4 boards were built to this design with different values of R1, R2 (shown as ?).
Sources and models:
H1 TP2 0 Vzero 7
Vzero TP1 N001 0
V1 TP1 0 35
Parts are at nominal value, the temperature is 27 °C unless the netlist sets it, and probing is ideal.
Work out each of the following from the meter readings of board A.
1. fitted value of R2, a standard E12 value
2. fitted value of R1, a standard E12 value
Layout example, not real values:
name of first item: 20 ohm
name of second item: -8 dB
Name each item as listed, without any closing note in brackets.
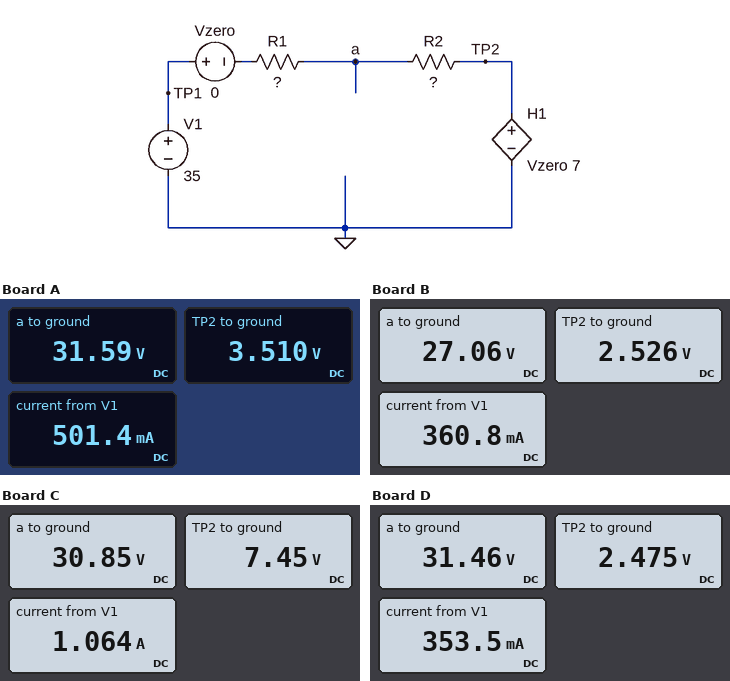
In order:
fitted value of R2, a standard E12 value: 56 Ω
fitted value of R1, a standard E12 value: 6.8 Ω
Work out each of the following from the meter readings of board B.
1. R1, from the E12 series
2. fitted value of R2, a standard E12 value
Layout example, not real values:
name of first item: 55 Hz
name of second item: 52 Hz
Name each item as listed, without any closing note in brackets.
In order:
R1, from the E12 series: 22 Ω
fitted value of R2, a standard E12 value: 68 Ω
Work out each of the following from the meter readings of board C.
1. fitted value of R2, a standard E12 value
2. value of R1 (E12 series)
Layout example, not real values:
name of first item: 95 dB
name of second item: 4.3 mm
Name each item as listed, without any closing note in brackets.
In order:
fitted value of R2, a standard E12 value: 22 Ω
value of R1: 3.9 Ω
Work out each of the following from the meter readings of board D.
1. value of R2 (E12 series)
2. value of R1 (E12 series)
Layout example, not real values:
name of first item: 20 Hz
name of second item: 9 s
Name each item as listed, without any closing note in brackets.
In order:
value of R2: 82 Ω
value of R1: 10 Ω
